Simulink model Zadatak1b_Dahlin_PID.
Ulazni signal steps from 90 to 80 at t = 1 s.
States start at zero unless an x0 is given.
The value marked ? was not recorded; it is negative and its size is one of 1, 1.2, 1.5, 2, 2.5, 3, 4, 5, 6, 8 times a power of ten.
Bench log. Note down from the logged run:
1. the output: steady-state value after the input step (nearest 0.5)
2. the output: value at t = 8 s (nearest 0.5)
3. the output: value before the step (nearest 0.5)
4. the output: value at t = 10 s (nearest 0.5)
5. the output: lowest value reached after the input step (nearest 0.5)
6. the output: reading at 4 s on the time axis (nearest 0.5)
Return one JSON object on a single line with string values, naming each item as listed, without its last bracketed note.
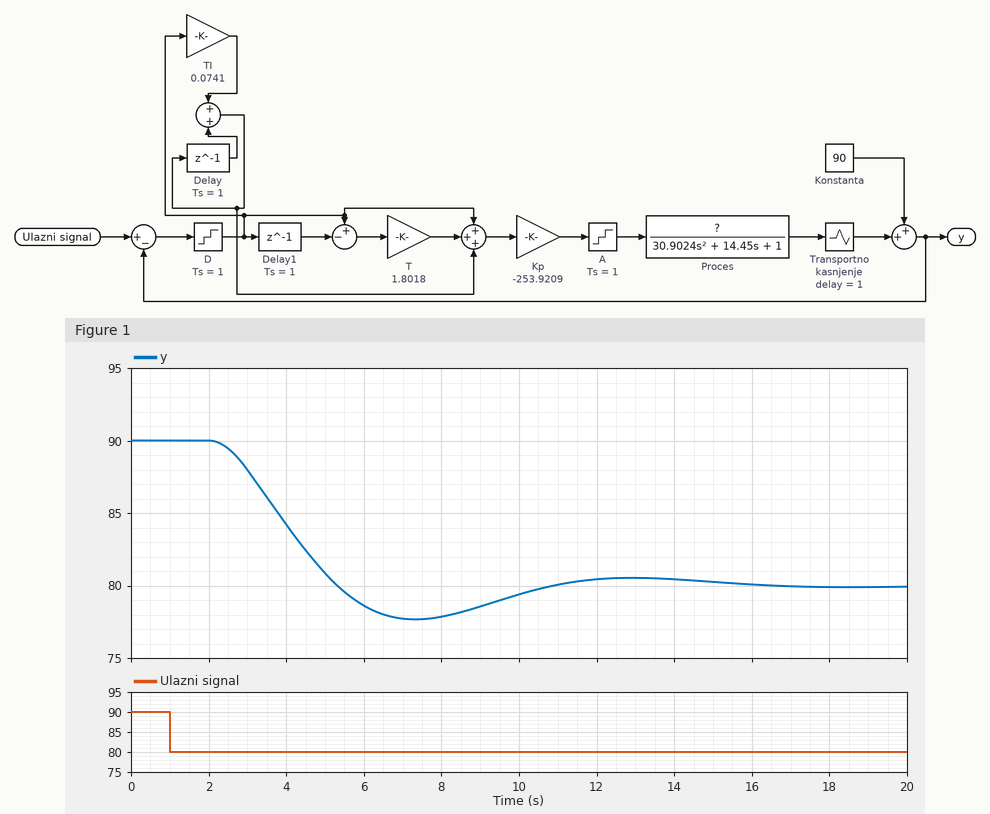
{"the output: steady-state value after the input step": "80.0", "the output: value at t = 8 s": "78.0", "the output: value before the step": "90.0", "the output: value at t = 10 s": "79.5", "the output: lowest value reached after the input step": "77.5", "the output: reading at 4 s on the time axis": "84.0"}
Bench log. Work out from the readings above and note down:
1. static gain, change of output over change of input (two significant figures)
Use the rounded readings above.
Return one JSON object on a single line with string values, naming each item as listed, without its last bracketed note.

{"static gain, change of output over change of input": "1.0"}
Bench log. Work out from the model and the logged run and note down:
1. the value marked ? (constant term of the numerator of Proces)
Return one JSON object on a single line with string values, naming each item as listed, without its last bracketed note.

{"the value marked ?": "-0.02"}
